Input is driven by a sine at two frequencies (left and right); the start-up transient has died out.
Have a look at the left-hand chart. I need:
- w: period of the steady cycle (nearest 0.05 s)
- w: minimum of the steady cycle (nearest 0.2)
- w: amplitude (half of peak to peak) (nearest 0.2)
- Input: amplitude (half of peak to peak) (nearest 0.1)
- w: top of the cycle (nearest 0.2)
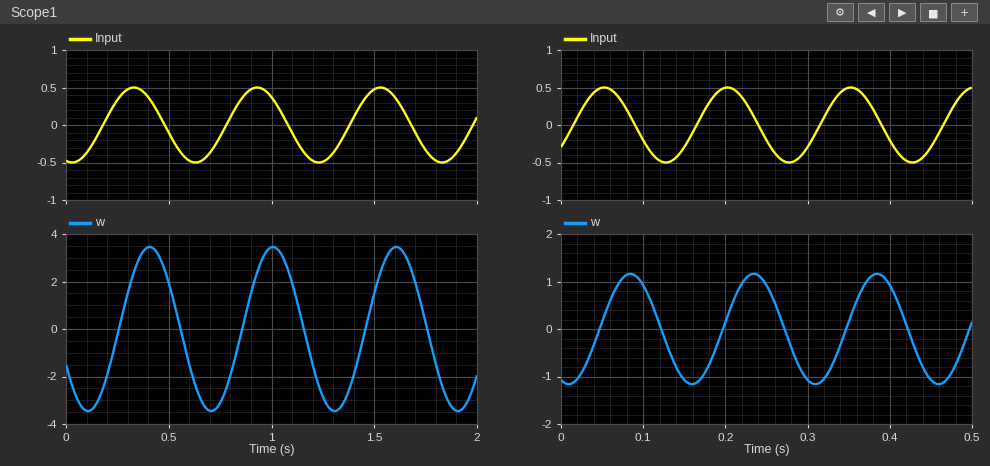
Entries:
0.60 s
-3.4
3.4
0.5
3.4
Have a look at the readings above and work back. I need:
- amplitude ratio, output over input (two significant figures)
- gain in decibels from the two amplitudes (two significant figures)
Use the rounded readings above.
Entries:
6.8
17 dB
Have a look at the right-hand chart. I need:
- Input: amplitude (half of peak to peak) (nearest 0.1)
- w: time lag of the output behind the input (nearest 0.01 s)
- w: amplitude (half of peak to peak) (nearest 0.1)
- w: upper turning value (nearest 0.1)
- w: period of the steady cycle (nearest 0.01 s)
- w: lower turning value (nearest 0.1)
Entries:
0.5
0.03 s
1.2
1.2
0.15 s
-1.2
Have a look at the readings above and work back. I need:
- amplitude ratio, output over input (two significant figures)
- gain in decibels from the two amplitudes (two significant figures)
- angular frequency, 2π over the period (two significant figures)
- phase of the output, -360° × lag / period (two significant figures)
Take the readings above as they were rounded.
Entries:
2.4
7.6 dB
42 rad/s
-72°
